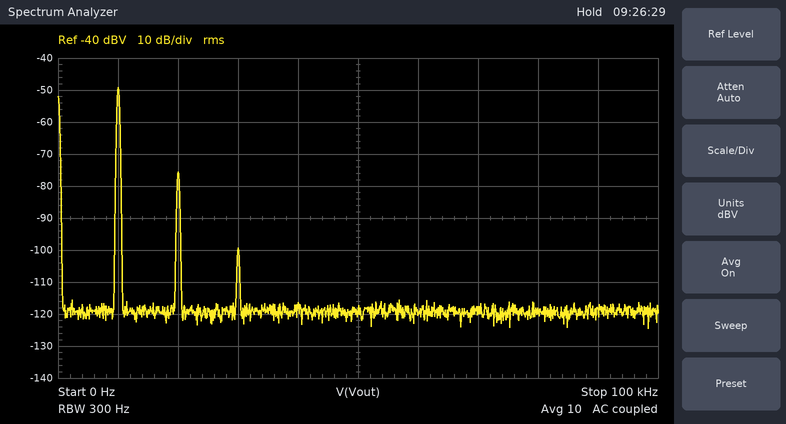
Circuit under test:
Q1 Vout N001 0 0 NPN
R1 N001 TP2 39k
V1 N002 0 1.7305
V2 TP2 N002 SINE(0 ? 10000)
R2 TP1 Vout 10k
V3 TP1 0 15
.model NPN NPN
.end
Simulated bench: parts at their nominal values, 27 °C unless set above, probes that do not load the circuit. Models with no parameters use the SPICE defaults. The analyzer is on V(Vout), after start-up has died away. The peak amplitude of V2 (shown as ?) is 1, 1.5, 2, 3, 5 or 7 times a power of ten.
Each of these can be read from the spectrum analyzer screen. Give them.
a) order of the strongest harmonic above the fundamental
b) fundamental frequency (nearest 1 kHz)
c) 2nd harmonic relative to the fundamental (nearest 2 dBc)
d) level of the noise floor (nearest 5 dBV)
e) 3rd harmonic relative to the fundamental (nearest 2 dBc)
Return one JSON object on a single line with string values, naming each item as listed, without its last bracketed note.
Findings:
{"order of the strongest harmonic above the fundamental": "2", "fundamental frequency": "10 kHz", "2nd harmonic relative to the fundamental": "-26 dBc", "level of the noise floor": "-120 dBV", "3rd harmonic relative to the fundamental": "-50 dBc"}
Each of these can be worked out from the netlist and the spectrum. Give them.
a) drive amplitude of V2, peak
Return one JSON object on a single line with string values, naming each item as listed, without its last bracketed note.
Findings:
{"drive amplitude of V2, peak": "70 mV"}
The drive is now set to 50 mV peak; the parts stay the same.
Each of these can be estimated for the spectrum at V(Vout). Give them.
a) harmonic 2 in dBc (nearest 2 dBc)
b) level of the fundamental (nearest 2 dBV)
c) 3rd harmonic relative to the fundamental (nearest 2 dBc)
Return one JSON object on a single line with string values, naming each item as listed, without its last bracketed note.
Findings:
{"harmonic 2 in dBc": "-30 dBc", "level of the fundamental": "-52 dBV", "3rd harmonic relative to the fundamental": "-56 dBc"}
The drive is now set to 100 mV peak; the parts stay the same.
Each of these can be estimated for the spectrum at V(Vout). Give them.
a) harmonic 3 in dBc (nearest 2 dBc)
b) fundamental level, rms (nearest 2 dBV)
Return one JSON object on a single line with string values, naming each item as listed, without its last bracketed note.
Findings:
{"harmonic 3 in dBc": "-44 dBc", "fundamental level, rms": "-46 dBV"}
